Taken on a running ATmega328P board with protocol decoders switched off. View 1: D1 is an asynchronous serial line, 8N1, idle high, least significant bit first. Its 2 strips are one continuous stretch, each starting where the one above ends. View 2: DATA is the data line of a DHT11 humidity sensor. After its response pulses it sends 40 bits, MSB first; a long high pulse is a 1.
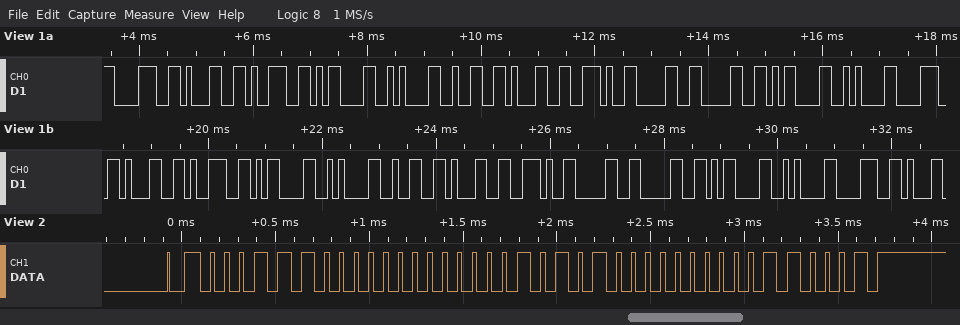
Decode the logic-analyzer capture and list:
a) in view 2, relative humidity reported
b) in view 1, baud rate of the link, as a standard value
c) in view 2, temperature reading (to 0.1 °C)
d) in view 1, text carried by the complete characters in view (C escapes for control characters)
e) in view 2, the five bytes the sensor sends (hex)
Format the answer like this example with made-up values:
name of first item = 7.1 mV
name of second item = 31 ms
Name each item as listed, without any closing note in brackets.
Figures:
in view 2, relative humidity reported = 28 %
in view 1, baud rate of the link, as a standard value = 9600 baud
in view 2, temperature reading = 21.0 °C
in view 1, text carried by the complete characters in view = "819\r\n21.00\r\n819\r\n21.00\r\n8"
in view 2, the five bytes the sensor sends = 1C 00 15 00 31
